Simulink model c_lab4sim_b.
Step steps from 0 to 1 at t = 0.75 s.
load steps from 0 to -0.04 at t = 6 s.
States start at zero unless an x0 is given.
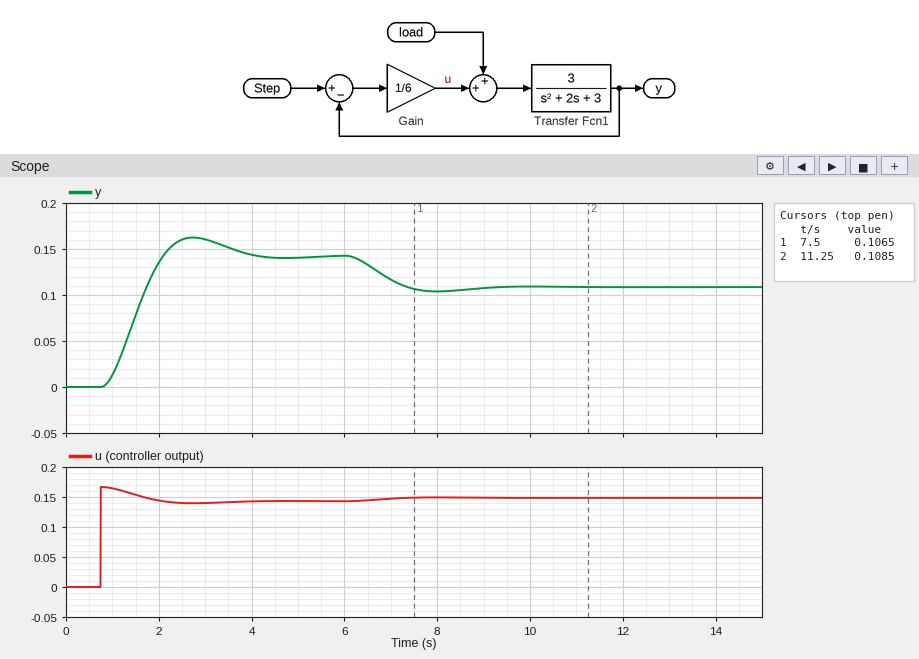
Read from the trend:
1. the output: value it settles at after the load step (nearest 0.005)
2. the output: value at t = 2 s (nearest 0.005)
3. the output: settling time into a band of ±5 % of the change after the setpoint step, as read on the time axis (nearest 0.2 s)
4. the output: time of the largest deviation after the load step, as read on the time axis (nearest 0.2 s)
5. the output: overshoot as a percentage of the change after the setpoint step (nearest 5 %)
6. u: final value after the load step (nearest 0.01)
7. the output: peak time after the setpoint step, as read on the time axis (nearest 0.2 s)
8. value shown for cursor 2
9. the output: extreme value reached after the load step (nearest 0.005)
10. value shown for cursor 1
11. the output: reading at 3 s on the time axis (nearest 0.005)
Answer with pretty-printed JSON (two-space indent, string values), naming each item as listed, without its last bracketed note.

{
  "the output: value it settles at after the load step": "0.110",
  "the output: value at t = 2 s": "0.135",
  "the output: settling time into a band of ±5 % of the change after the setpoint step, as read on the time axis": "3.6 s",
  "the output: time of the largest deviation after the load step, as read on the time axis": "8.0 s",
  "the output: overshoot as a percentage of the change after the setpoint step": "15 %",
  "u: final value after the load step": "0.15",
  "the output: peak time after the setpoint step, as read on the time axis": "2.8 s",
  "value shown for cursor 2": "0.1085",
  "the output: extreme value reached after the load step": "0.105",
  "value shown for cursor 1": "0.1065",
  "the output: reading at 3 s on the time axis": "0.160"
}
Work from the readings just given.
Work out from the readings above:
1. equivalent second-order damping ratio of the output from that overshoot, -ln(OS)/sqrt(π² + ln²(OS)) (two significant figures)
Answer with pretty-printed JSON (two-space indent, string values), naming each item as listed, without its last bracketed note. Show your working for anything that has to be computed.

{
  "equivalent second-order damping ratio of the output from that overshoot, -ln(OS)/sqrt(π² + ln²(OS))": "ln(0.15) = -1.897; 1.897 / sqrt(9.870 + 3.599) = 0.52"
}
